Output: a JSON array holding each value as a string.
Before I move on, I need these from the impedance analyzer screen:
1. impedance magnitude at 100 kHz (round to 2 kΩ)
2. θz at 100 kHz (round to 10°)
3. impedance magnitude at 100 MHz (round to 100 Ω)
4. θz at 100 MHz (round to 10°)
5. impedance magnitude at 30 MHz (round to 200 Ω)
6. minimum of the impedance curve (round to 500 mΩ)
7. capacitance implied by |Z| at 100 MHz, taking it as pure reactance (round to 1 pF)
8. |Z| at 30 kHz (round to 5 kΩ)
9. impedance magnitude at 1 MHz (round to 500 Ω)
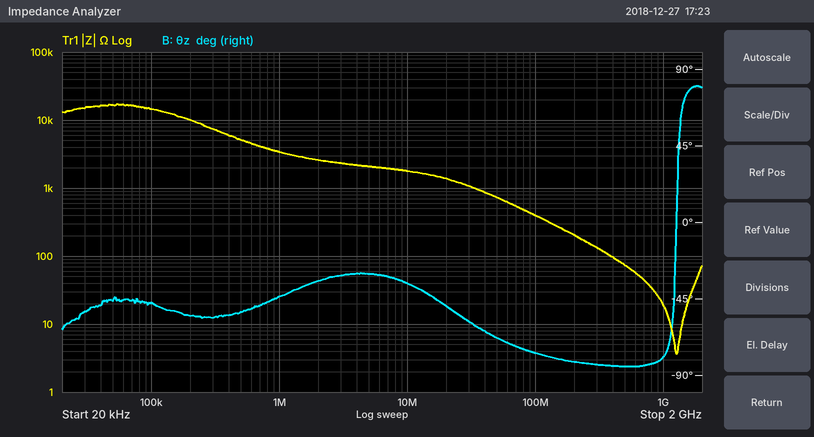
["14 kΩ", "-50°", "400 Ω", "-80°", "1.0 kΩ", "3.5 Ω", "4 pF", "15 kΩ", "3.5 kΩ"]
